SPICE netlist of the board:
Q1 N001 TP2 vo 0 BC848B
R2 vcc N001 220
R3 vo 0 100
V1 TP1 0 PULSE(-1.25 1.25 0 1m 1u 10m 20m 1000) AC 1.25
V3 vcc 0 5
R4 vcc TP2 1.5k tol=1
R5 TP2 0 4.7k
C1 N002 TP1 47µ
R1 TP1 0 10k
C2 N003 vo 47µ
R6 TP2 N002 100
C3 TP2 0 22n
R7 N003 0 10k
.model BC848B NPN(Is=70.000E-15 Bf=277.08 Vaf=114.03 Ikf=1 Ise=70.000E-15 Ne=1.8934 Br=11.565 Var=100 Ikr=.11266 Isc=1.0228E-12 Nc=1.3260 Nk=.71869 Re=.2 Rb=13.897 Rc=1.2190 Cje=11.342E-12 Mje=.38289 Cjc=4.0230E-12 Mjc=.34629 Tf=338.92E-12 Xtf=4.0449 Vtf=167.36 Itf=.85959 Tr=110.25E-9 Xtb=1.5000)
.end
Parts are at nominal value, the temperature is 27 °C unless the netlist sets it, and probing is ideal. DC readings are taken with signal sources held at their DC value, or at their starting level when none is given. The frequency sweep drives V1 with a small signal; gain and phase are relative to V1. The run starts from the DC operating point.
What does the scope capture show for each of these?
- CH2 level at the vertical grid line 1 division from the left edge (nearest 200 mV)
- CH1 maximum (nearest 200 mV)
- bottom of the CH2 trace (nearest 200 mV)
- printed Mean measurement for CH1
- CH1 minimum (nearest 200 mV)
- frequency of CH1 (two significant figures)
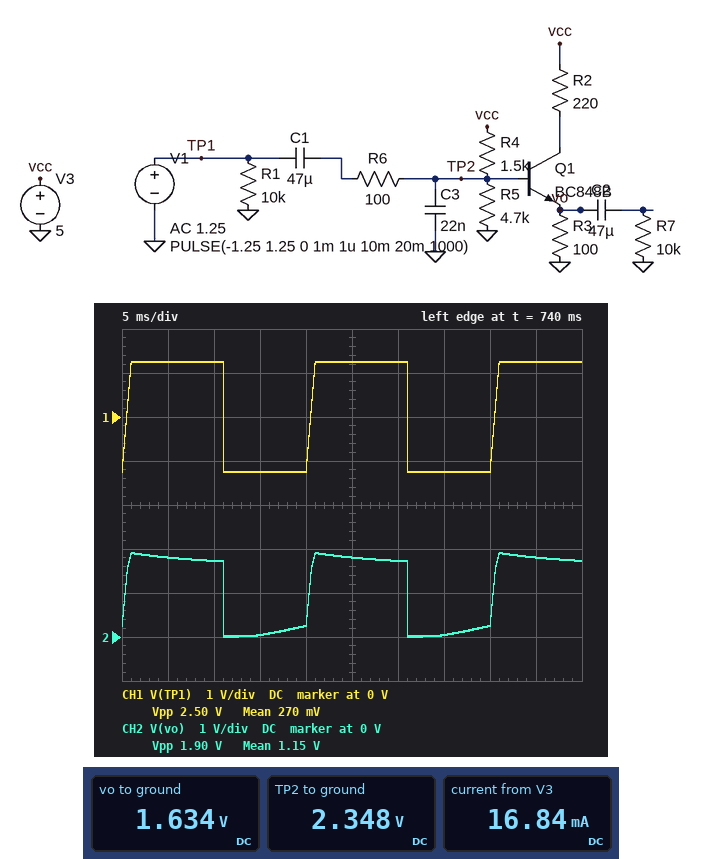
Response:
1.8 V
1.2 V
0 V
270 mV
-1.2 V
50 Hz
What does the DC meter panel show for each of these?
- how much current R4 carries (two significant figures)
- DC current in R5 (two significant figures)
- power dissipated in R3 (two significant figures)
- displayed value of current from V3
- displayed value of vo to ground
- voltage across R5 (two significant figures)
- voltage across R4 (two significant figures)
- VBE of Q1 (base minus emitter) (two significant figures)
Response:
1.8 mA
500 µA
27 mW
16.84 mA
1.634 V
2.3 V
2.7 V
710 mV
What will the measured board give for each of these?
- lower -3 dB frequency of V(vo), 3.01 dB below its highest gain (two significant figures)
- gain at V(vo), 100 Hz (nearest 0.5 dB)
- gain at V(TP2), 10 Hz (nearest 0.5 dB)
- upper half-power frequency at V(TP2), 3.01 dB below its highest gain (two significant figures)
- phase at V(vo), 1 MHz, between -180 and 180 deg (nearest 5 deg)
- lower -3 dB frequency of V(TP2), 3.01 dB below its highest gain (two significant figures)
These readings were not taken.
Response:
18 Hz
-9.0 dB
-13.0 dB
140 kHz
-80 deg
18 Hz
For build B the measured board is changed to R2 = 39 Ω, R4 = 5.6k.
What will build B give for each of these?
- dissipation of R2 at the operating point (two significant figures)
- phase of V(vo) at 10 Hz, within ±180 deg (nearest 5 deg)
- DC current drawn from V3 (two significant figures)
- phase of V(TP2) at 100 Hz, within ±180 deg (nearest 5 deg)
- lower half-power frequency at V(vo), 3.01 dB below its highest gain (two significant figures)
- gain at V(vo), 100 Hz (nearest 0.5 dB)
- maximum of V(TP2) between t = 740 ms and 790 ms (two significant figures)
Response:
8.3 mW
10 deg
15 mA
0 deg
1.4 Hz
-0.5 dB
3.3 V
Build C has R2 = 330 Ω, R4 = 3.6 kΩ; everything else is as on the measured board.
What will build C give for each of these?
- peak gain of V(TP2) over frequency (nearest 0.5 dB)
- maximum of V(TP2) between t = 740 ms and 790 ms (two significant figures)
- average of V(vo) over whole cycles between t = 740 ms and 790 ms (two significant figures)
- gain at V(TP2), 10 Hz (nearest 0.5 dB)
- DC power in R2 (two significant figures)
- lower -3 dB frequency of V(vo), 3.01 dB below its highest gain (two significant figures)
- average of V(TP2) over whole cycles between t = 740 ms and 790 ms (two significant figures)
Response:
-5.5 dB
2.1 V
680 mV
-11.0 dB
43 mW
16 Hz
980 mV
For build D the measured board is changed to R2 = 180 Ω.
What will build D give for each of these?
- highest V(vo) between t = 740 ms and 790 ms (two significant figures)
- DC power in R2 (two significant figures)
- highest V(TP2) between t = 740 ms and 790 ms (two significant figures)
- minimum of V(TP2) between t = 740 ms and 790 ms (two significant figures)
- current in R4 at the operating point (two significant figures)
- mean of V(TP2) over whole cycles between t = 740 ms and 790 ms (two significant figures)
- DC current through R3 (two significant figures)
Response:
2.1 V
54 mW
2.9 V
560 mV
1.6 mA
1.8 V
18 mA
